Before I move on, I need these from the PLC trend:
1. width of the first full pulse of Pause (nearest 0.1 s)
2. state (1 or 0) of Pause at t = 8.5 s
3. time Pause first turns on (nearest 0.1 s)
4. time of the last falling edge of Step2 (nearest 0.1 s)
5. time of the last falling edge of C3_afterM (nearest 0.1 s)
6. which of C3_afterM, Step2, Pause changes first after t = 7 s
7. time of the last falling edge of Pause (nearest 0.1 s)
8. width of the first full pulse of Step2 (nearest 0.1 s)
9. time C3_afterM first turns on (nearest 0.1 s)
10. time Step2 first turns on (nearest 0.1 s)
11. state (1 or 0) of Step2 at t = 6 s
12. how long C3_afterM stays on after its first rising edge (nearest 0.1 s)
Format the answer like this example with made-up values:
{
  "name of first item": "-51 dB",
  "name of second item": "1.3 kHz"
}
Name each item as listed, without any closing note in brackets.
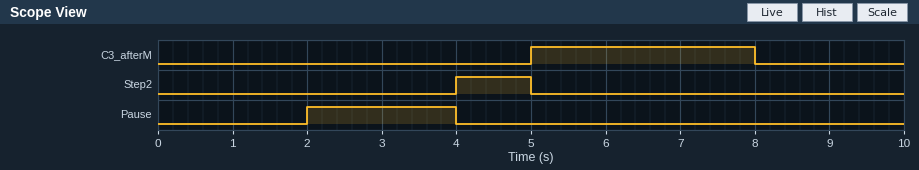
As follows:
{
  "width of the first full pulse of Pause": "2.0 s",
  "state (1 or 0) of Pause at t = 8.5 s": "0",
  "time Pause first turns on": "2.0 s",
  "time of the last falling edge of Step2": "5.0 s",
  "time of the last falling edge of C3_afterM": "8.0 s",
  "which of C3_afterM, Step2, Pause changes first after t = 7 s": "C3_afterM",
  "time of the last falling edge of Pause": "4.0 s",
  "width of the first full pulse of Step2": "1.0 s",
  "time C3_afterM first turns on": "5.0 s",
  "time Step2 first turns on": "4.0 s",
  "state (1 or 0) of Step2 at t = 6 s": "0",
  "how long C3_afterM stays on after its first rising edge": "3.0 s"
}
